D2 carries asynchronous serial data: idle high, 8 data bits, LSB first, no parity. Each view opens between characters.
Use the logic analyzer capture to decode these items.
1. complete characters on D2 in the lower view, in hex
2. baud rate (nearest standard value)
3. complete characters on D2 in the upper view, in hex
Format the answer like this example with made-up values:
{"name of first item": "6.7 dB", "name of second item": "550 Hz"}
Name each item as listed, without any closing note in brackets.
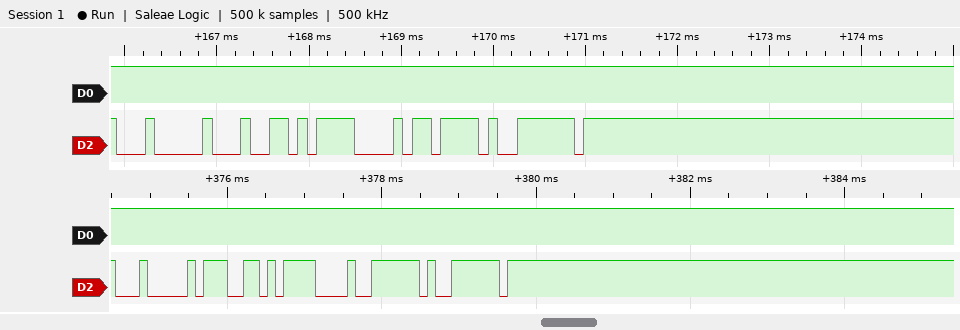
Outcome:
{"complete characters on D2 in the lower view, in hex": "04, 67, 0F, 7E, 7E", "baud rate": "9600 baud", "complete characters on D2 in the upper view, in hex": "04, 64, 0F, 7B, 7E"}
